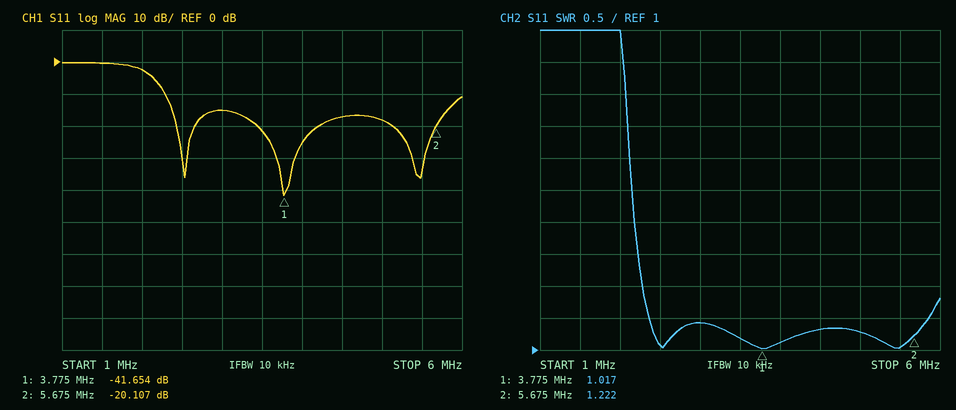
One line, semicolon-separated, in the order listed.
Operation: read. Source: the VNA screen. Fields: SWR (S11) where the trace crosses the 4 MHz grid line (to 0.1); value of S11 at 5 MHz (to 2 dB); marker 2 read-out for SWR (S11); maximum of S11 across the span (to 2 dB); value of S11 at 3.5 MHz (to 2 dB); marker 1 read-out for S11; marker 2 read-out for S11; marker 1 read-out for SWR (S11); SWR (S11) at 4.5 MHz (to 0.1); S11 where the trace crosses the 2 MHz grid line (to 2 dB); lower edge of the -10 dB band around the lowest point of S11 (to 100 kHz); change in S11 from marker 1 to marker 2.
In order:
1.1; -18 dB; 1.222; 0 dB; -22 dB; -41.654 dB; -20.107 dB; 1.017; 1.3; -2 dB; 2.3 MHz; 21.547 dB
